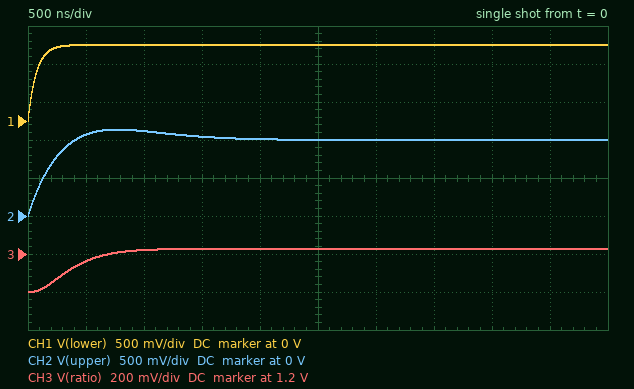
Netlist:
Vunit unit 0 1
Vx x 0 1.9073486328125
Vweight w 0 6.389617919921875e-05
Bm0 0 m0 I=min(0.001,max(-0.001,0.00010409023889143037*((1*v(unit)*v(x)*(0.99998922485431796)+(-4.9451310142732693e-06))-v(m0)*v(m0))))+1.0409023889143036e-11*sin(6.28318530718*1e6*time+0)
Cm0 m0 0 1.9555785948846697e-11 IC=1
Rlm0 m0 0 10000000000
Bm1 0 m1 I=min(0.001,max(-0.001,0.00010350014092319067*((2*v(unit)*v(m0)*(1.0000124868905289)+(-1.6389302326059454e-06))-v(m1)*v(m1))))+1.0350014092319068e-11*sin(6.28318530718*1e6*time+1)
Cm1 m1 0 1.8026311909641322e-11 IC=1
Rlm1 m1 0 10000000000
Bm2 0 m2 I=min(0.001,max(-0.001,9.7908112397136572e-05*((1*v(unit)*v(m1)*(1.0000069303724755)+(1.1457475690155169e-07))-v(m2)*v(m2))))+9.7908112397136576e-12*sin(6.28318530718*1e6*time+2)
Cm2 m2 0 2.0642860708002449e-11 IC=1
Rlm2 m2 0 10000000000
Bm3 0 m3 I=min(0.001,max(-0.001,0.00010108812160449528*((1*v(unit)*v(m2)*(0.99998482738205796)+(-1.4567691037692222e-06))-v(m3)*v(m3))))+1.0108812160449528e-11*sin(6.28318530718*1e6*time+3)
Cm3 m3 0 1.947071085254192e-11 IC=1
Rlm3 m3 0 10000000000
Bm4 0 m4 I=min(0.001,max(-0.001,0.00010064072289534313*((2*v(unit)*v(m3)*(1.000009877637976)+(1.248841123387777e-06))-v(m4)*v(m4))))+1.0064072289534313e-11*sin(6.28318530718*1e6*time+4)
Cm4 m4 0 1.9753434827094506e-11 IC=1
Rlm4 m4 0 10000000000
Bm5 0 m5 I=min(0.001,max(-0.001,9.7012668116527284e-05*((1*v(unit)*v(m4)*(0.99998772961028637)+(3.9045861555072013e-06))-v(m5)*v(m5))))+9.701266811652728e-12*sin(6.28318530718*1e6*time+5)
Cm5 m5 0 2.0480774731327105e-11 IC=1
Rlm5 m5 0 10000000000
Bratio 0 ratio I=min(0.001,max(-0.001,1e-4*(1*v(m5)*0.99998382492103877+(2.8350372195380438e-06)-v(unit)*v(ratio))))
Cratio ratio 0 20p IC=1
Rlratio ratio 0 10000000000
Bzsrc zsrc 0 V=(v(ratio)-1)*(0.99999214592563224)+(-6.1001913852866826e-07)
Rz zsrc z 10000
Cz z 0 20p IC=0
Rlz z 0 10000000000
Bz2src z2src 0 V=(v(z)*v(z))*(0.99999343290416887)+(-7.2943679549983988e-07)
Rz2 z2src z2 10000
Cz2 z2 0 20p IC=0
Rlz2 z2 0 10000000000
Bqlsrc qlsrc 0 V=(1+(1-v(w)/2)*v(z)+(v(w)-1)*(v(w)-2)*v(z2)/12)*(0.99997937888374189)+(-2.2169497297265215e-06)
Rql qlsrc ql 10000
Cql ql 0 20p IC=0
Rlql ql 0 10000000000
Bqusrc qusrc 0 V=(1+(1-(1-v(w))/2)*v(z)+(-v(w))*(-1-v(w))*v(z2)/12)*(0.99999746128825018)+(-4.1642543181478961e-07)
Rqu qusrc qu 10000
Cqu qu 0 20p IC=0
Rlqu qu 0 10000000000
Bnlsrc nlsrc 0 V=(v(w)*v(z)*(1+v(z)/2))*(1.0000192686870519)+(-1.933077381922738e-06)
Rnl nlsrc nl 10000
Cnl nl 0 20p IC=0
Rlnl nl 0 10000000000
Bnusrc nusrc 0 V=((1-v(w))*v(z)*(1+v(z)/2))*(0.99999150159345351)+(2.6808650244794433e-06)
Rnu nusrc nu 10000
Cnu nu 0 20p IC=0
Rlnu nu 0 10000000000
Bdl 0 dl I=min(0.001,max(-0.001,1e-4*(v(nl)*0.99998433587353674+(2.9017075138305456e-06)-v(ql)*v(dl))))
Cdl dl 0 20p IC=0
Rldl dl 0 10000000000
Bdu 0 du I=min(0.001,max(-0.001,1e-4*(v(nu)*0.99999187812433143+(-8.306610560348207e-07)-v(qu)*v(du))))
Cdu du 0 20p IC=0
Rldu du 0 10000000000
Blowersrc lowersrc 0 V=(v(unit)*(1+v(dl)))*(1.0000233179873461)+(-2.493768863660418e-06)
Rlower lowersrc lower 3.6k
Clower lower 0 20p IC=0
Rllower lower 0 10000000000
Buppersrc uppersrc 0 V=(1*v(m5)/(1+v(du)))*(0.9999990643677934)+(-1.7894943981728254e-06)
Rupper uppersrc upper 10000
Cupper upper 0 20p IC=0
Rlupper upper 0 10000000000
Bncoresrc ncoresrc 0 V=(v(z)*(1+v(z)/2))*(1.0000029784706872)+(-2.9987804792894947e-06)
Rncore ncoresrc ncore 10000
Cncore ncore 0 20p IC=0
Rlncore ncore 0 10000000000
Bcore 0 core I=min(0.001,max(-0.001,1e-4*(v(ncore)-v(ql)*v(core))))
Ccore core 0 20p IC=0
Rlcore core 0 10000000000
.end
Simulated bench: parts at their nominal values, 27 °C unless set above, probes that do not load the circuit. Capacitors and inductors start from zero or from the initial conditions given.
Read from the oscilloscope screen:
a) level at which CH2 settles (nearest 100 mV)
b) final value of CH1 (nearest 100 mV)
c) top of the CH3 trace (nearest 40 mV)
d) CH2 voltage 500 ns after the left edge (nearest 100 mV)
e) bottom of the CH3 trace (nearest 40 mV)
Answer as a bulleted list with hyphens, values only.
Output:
- 1.0 V
- 1.0 V
- 1.24 V
- 1.1 V
- 1.00 V
